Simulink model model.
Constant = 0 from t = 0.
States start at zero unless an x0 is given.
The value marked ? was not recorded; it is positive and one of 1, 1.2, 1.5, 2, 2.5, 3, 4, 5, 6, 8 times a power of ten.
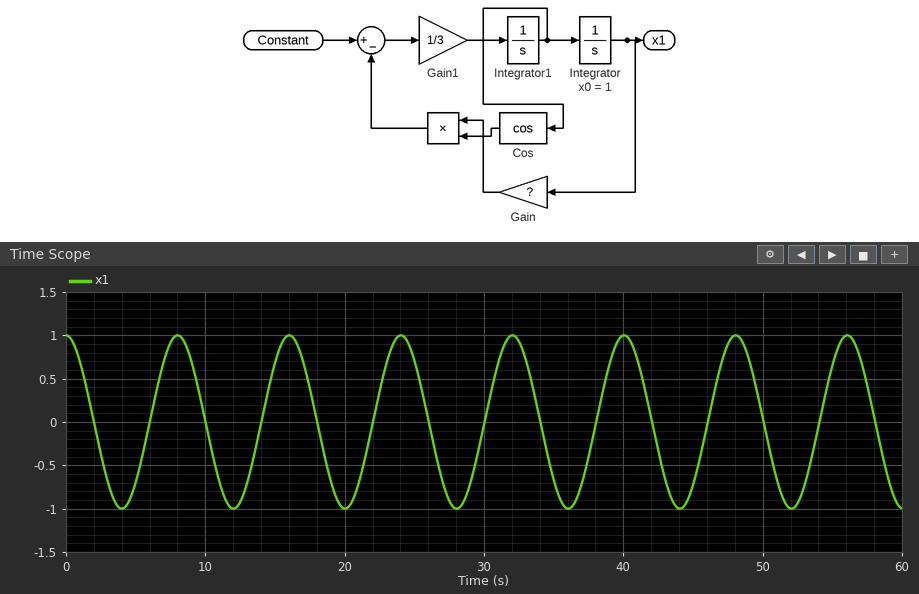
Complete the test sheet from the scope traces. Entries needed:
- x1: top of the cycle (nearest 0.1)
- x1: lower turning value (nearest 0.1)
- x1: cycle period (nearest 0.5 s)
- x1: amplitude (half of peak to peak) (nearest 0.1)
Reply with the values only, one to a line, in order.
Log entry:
1.0
-1.0
8.0 s
1.0
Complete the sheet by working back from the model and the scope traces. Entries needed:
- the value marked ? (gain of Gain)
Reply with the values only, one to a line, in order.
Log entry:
2
